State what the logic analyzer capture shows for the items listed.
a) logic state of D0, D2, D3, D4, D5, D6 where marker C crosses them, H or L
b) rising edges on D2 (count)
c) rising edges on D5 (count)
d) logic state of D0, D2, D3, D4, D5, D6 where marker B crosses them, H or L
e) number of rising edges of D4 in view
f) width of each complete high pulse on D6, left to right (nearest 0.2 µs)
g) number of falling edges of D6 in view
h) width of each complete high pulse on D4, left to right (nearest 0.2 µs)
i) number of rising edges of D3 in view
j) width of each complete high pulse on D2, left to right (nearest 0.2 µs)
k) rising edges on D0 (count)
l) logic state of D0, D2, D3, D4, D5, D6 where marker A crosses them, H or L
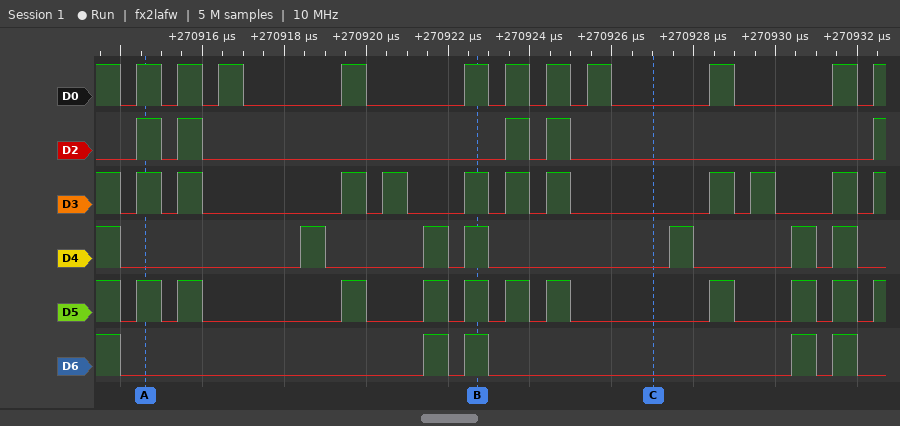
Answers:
D0=L, D2=L, D3=L, D4=L, D5=L, D6=L
5
11
D0=H, D2=L, D3=H, D4=H, D5=H, D6=H
6
0.6 µs, 0.6 µs, 0.6 µs, 0.6 µs
5
0.6 µs, 0.6 µs, 0.6 µs, 0.6 µs, 0.6 µs, 0.6 µs
11
0.6 µs, 0.6 µs, 0.6 µs, 0.6 µs
11
D0=H, D2=H, D3=H, D4=L, D5=H, D6=L
